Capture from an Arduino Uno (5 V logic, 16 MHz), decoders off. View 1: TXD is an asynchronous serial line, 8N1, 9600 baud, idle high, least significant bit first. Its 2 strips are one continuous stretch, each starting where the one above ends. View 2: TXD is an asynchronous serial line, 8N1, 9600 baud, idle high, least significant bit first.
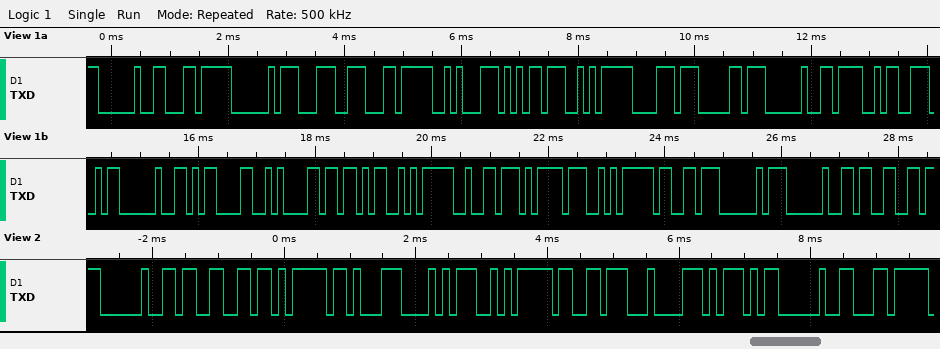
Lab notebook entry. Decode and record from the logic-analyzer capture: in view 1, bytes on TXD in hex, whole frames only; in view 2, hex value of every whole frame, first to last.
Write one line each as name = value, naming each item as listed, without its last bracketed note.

in view 1, bytes on TXD in hex, whole frames only = 0x20 0xEC 0xA0 0x9C 0xEC 0x8A 0xB5 0xEA 0xB8 0xB0 0x20 0x4F 0x4E 0x20 0x0D 0x0A 0x5B 0xEA 0xB2 0xBD 0xEA 0xB3 0xA0 0x20 0x33
in view 2, hex value of every whole frame, first to last = 0x20 0x33 0xEB 0x8B 0xA8 0xEA 0xB3 0x84 0x5D 0x20 0xEC
